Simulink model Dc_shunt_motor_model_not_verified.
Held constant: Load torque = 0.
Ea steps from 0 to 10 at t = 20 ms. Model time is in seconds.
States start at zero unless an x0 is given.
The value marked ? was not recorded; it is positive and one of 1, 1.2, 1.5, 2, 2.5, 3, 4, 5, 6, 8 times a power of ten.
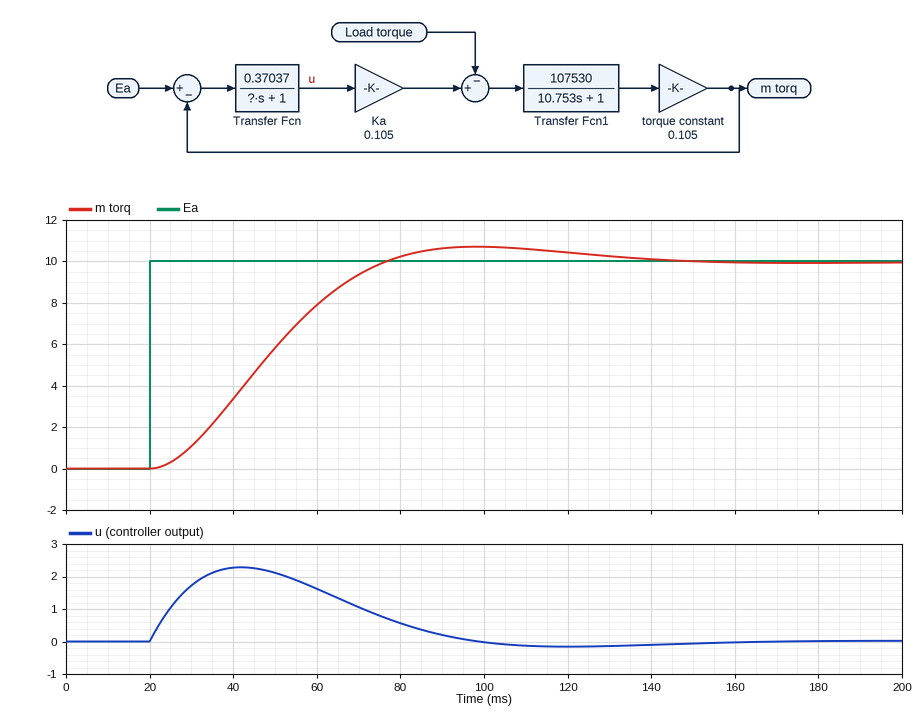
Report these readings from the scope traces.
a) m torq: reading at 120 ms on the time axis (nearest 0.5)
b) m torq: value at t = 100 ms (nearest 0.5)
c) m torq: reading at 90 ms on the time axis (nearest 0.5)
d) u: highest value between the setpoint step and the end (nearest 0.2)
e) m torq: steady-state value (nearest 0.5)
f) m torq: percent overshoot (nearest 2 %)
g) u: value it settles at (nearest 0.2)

10.5
10.5
10.5
2.2
10.0
8 %
0.0
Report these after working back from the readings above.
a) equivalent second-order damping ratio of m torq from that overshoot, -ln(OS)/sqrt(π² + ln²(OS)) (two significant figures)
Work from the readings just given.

0.63
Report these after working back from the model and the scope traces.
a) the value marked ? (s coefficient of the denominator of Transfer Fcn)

0.015
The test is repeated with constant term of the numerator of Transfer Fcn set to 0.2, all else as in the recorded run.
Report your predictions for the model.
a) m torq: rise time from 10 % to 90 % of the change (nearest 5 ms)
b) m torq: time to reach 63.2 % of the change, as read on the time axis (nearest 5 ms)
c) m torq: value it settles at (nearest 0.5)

70 ms
70 ms
10.0
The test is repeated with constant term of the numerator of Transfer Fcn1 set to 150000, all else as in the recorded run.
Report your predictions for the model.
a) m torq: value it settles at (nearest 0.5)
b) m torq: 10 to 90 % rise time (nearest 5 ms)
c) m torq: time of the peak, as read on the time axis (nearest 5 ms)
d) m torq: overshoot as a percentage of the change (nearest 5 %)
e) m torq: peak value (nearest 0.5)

10.0
30 ms
80 ms
15 %
11.5
